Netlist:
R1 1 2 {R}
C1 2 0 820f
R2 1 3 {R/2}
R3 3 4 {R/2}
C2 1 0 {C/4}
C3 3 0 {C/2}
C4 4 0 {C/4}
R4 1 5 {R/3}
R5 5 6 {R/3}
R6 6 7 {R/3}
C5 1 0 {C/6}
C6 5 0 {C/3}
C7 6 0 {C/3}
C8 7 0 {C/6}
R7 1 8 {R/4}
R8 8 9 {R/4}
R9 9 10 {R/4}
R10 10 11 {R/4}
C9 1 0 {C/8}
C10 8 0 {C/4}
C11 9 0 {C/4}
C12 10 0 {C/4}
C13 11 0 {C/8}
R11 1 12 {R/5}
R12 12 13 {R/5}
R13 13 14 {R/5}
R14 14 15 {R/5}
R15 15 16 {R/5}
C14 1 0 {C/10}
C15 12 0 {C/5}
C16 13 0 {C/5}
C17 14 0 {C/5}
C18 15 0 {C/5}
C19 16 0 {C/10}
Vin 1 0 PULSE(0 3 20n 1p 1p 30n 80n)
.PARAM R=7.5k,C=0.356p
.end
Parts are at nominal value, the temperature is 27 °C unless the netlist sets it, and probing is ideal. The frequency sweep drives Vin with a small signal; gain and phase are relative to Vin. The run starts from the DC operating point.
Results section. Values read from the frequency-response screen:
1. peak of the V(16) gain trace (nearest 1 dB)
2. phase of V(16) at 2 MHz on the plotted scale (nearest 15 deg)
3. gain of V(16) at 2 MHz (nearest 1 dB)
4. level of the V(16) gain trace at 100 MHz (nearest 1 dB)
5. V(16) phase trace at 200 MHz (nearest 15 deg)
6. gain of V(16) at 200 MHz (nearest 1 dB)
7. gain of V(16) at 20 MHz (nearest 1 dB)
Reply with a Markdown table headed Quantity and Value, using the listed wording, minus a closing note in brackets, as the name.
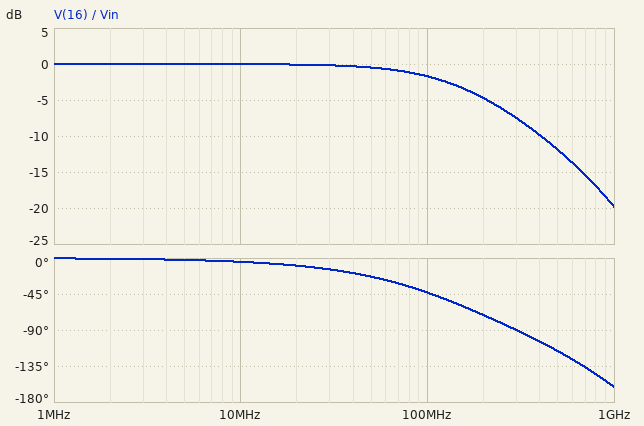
| Quantity | Value |
|---|---|
| peak of the V(16) gain trace | 0 dB |
| phase of V(16) at 2 MHz on the plotted scale | 0 deg |
| gain of V(16) at 2 MHz | 0 dB |
| level of the V(16) gain trace at 100 MHz | -2 dB |
| V(16) phase trace at 200 MHz | -75 deg |
| gain of V(16) at 200 MHz | -5 dB |
| gain of V(16) at 20 MHz | 0 dB |
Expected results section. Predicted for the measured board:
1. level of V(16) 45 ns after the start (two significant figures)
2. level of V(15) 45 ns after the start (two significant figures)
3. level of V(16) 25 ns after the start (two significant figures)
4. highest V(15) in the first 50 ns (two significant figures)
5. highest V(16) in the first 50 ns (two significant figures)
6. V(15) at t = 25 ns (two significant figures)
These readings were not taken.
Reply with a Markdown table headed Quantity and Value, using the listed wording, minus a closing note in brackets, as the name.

| Quantity | Value |
|---|---|
| level of V(16) 45 ns after the start | 3.0 V |
| level of V(15) 45 ns after the start | 3.0 V |
| level of V(16) 25 ns after the start | 3.0 V |
| highest V(15) in the first 50 ns | 3.0 V |
| highest V(16) in the first 50 ns | 3.0 V |
| V(15) at t = 25 ns | 3.0 V |
